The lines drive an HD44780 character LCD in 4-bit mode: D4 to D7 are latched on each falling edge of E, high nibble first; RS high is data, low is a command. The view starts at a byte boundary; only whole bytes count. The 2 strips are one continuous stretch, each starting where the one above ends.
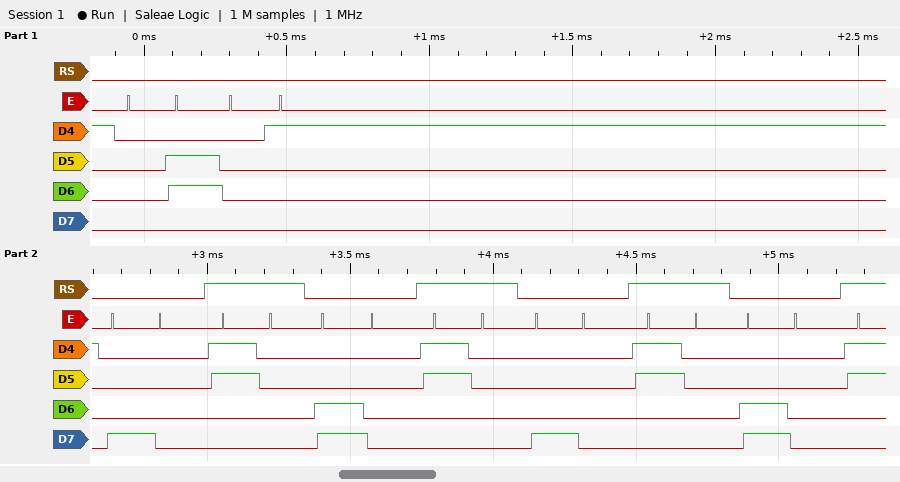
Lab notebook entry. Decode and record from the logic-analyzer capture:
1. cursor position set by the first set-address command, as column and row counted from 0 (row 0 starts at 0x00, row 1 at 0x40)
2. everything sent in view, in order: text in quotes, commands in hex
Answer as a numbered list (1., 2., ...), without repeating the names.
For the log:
1. column 0, row 0
2. 0x06 0x01 0x80 "0" 0xC0 "0" 0x80 "0" 0xC0
